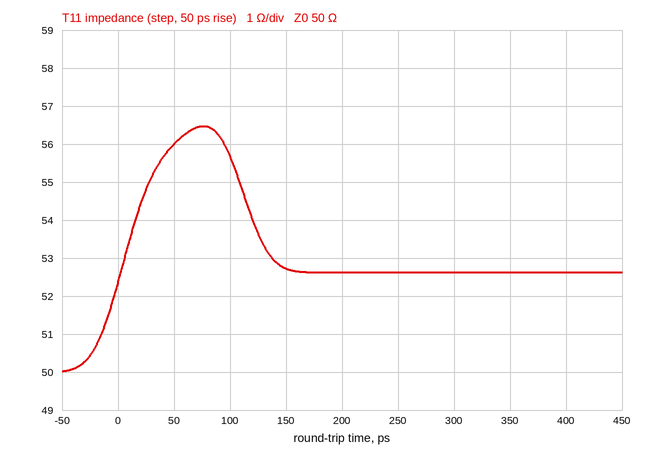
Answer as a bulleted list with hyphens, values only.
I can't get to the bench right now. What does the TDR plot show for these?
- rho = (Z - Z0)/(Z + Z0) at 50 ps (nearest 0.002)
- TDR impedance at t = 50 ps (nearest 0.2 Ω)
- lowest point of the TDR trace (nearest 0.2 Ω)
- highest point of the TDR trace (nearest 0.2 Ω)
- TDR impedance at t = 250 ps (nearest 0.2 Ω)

- +0.056
- 56.0 Ω
- 50.0 Ω
- 56.4 Ω
- 52.6 Ω
